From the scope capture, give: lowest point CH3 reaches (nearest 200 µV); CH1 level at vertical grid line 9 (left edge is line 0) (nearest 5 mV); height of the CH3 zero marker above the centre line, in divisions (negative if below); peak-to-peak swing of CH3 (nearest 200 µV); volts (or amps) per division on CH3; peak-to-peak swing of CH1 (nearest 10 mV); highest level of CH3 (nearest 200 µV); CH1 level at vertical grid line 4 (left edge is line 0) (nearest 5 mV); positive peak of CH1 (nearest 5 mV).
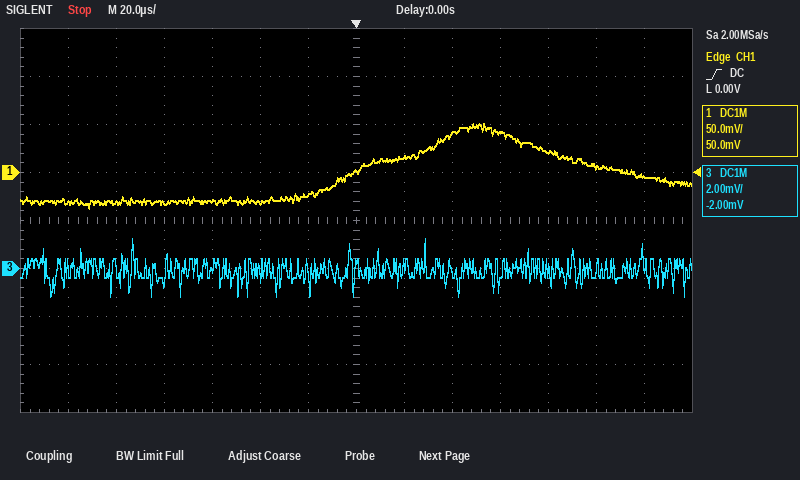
-1.2 mV
40 mV
-1.0 div
2.4 mV
2 mV
90 mV
1.2 mV
-30 mV
50 mV
